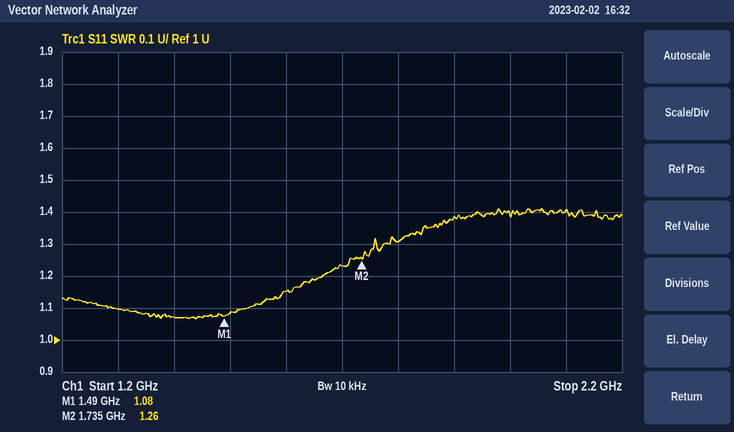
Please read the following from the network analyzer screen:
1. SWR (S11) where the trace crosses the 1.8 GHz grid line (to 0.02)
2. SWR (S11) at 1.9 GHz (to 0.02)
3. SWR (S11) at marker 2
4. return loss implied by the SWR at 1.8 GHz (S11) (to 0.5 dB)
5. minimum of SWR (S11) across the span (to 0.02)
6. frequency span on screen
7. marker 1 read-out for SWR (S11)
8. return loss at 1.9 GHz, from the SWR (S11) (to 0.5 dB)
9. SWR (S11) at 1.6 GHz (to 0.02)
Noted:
1.30
1.38
1.26
17.5 dB
1.06
1 GHz
1.08
16.0 dB
1.16
